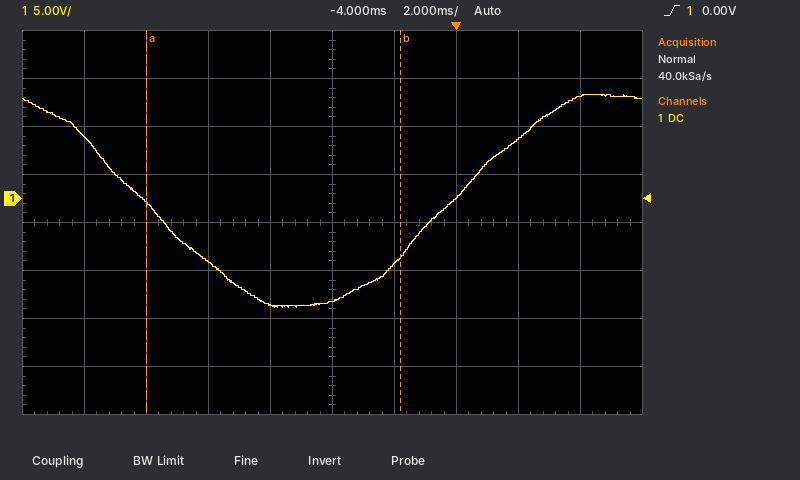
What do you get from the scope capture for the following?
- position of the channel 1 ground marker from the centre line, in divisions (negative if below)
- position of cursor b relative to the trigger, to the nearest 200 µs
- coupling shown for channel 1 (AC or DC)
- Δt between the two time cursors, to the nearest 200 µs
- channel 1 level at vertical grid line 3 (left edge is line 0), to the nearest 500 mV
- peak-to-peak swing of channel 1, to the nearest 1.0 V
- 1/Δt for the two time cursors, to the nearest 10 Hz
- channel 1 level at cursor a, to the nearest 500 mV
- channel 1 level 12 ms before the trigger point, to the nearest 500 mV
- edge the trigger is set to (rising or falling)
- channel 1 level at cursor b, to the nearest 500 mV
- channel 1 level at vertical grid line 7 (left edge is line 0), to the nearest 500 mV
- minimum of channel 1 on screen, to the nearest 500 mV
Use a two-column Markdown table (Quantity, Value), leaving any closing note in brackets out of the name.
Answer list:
| Quantity | Value |
|---|---|
| position of the channel 1 ground marker from the centre line, in divisions | +0.5 div |
| position of cursor b relative to the trigger, to the nearest 200 µs | -1.8 ms |
| coupling shown for channel 1 | DC |
| Δt between the two time cursors, to the nearest 200 µs | 8.2 ms |
| channel 1 level at vertical grid line 3 (left edge is line 0), to the nearest 500 mV | -6.5 V |
| peak-to-peak swing of channel 1, to the nearest 1.0 V | 22.0 V |
| 1/Δt for the two time cursors, to the nearest 10 Hz | 120 Hz |
| channel 1 level at cursor a, to the nearest 500 mV | -500 mV |
| channel 1 level 12 ms before the trigger point, to the nearest 500 mV | 6.5 V |
| edge the trigger is set to | rising |
| channel 1 level at cursor b, to the nearest 500 mV | -6.0 V |
| channel 1 level at vertical grid line 7 (left edge is line 0), to the nearest 500 mV | 0.0 V |
| minimum of channel 1 on screen, to the nearest 500 mV | -11.5 V |
